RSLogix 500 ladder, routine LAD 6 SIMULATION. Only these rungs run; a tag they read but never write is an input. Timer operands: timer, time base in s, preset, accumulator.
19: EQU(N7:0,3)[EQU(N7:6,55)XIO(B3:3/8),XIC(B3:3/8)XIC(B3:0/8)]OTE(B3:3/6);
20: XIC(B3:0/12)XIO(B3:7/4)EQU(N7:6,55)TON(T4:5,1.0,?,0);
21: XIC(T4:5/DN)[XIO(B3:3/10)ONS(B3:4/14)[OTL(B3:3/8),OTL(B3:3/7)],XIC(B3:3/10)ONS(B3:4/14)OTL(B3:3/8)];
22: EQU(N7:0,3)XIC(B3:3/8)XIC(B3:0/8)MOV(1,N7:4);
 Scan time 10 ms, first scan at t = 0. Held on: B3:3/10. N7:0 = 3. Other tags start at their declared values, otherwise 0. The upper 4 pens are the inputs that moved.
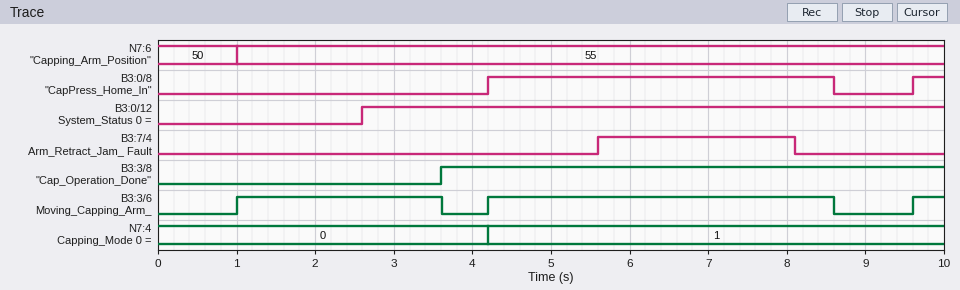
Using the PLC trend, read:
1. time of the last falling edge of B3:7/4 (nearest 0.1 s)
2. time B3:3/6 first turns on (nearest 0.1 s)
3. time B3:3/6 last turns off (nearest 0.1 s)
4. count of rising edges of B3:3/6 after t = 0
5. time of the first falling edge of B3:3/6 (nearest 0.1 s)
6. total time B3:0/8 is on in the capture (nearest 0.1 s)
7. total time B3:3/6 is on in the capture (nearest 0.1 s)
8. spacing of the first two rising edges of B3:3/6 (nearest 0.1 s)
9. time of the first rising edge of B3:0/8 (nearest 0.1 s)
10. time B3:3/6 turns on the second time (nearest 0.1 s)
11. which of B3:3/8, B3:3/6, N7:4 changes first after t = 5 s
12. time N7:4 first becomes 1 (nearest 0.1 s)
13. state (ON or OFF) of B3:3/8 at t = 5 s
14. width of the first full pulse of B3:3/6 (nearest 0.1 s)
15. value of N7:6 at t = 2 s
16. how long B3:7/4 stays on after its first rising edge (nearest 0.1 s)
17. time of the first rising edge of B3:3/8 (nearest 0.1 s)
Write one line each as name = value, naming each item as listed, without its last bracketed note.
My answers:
time of the last falling edge of B3:7/4 = 8.1 s
time B3:3/6 first turns on = 1.0 s
time B3:3/6 last turns off = 8.6 s
count of rising edges of B3:3/6 after t = 0 = 3
time of the first falling edge of B3:3/6 = 3.6 s
total time B3:0/8 is on in the capture = 4.8 s
total time B3:3/6 is on in the capture = 7.4 s
spacing of the first two rising edges of B3:3/6 = 3.2 s
time of the first rising edge of B3:0/8 = 4.2 s
time B3:3/6 turns on the second time = 4.2 s
which of B3:3/8, B3:3/6, N7:4 changes first after t = 5 s = B3:3/6
time N7:4 first becomes 1 = 4.2 s
state (ON or OFF) of B3:3/8 at t = 5 s = ON
width of the first full pulse of B3:3/6 = 2.6 s
value of N7:6 at t = 2 s = 55
how long B3:7/4 stays on after its first rising edge = 2.5 s
time of the first rising edge of B3:3/8 = 3.6 s
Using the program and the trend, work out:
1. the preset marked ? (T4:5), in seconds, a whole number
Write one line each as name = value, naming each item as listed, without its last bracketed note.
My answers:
the preset marked ? (T4:5), in seconds, a whole number = 1 s
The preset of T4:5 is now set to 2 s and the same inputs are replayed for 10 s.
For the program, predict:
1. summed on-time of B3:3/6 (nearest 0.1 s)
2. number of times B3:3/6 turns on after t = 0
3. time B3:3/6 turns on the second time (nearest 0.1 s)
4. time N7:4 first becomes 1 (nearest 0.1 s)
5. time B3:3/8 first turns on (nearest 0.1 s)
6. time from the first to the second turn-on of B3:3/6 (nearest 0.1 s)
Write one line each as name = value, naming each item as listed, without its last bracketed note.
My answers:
summed on-time of B3:3/6 = 8.0 s
number of times B3:3/6 turns on after t = 0 = 2
time B3:3/6 turns on the second time = 9.6 s
time N7:4 first becomes 1 = 4.6 s
time B3:3/8 first turns on = 4.6 s
time from the first to the second turn-on of B3:3/6 = 8.6 s
